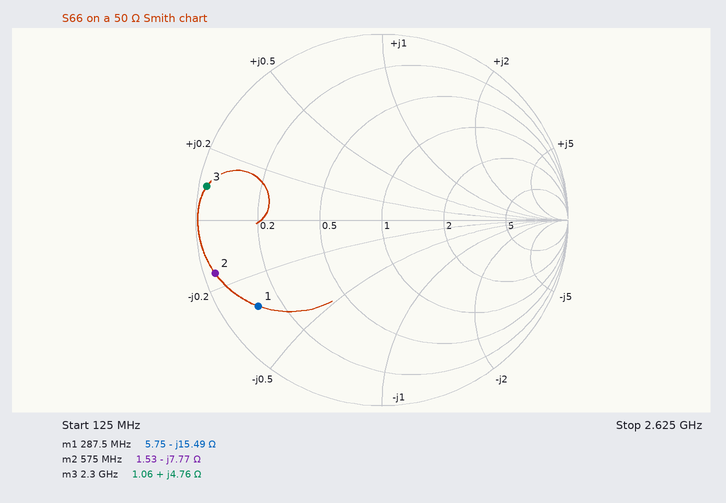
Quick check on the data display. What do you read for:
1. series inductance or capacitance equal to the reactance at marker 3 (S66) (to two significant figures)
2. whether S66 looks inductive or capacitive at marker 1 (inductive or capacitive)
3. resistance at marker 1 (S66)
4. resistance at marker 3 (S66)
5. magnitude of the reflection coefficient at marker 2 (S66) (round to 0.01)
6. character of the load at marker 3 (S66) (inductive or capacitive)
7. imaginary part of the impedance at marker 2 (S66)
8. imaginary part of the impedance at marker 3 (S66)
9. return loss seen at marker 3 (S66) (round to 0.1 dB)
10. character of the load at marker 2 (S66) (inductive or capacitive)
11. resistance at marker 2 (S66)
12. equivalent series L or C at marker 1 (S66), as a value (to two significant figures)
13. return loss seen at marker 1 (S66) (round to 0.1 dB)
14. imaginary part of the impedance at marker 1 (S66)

330 pH
capacitive
5.75 Ω
1.06 Ω
0.94
inductive
-7.77 Ω
+4.76 Ω
0.4 dB
capacitive
1.53 Ω
36 pF
1.8 dB
-15.49 Ω
